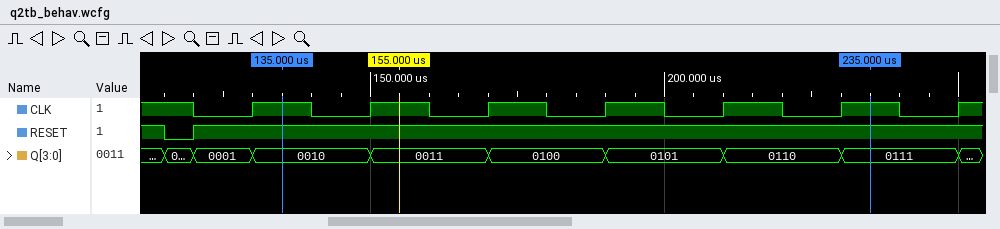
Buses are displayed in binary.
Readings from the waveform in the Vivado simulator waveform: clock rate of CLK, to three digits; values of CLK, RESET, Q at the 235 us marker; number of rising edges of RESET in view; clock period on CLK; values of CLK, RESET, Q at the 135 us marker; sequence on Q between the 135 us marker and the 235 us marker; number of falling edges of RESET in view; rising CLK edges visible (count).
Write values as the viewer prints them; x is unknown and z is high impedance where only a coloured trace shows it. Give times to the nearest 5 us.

50.0 kHz
CLK=1, RESET=1, Q=0111
1
20 us
CLK=1, RESET=1, Q=0010
0010, 0011, 0100, 0101, 0110, 0111
1
7
